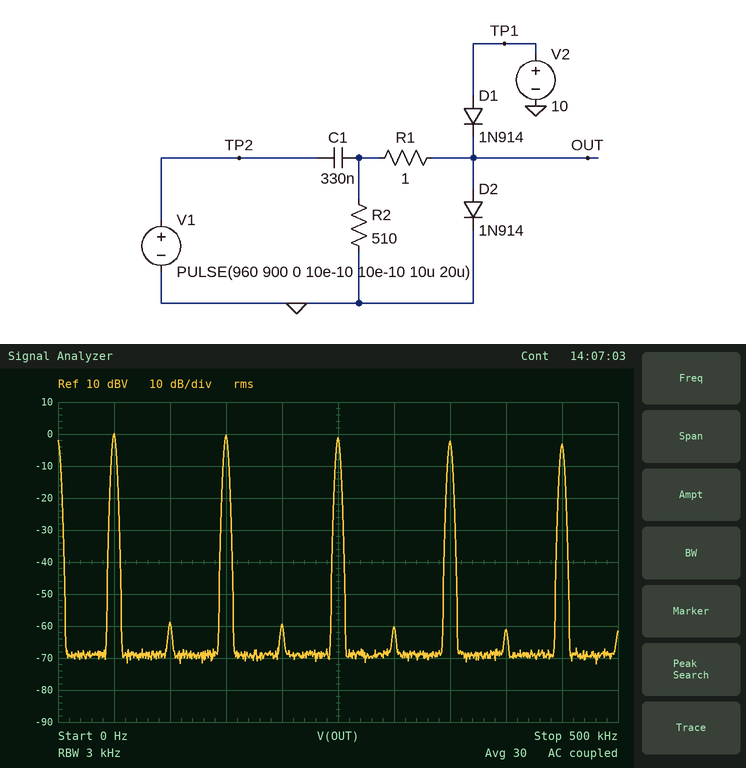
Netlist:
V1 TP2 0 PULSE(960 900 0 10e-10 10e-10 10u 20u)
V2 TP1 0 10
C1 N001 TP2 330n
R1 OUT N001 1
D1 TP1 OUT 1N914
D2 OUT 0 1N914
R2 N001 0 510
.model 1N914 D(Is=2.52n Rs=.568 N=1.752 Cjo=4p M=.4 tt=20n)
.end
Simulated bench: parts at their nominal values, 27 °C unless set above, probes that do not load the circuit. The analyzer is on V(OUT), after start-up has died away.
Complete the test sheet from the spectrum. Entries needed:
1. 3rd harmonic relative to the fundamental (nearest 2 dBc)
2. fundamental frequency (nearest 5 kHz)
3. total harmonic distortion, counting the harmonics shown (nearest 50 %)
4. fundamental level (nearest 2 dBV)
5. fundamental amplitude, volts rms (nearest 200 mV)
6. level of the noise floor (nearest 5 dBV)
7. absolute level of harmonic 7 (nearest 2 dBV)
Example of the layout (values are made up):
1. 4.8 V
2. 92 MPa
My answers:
1. 0 dBc
2. 50 kHz
3. 150 %
4. 0 dBV
5. 1.0 V
6. -70 dBV
7. -2 dBV
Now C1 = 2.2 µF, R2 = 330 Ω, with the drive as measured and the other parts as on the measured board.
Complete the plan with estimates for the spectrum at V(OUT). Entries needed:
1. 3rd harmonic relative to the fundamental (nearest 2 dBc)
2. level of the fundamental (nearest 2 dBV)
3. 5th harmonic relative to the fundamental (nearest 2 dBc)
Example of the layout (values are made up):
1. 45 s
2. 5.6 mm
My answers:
1. -6 dBc
2. 14 dBV
3. -10 dBc
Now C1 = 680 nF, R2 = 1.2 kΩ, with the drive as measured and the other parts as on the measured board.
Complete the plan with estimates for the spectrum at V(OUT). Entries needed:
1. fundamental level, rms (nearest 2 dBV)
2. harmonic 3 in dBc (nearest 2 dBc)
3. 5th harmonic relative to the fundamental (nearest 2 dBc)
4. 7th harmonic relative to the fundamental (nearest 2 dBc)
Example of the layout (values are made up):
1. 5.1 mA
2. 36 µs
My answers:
1. 6 dBV
2. -2 dBc
3. -4 dBc
4. -6 dBc
